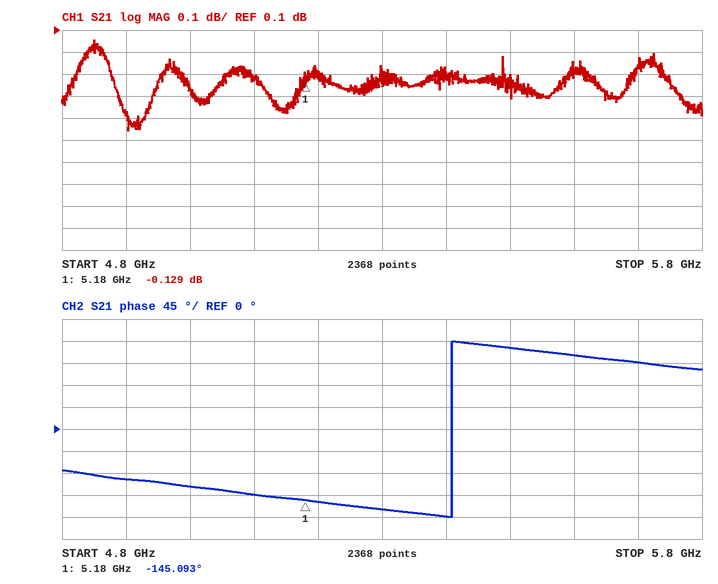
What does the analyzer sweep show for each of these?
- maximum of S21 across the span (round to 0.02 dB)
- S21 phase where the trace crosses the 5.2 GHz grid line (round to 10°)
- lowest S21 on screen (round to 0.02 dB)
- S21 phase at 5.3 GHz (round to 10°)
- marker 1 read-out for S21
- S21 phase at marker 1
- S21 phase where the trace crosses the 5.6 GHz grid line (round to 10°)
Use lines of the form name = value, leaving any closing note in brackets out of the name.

maximum of S21 across the span = 0.06 dB
S21 phase where the trace crosses the 5.2 GHz grid line = -150°
lowest S21 on screen = -0.36 dB
S21 phase at 5.3 GHz = -160°
marker 1 read-out for S21 = -0.129 dB
S21 phase at marker 1 = -145.093°
S21 phase where the trace crosses the 5.6 GHz grid line = 150°
